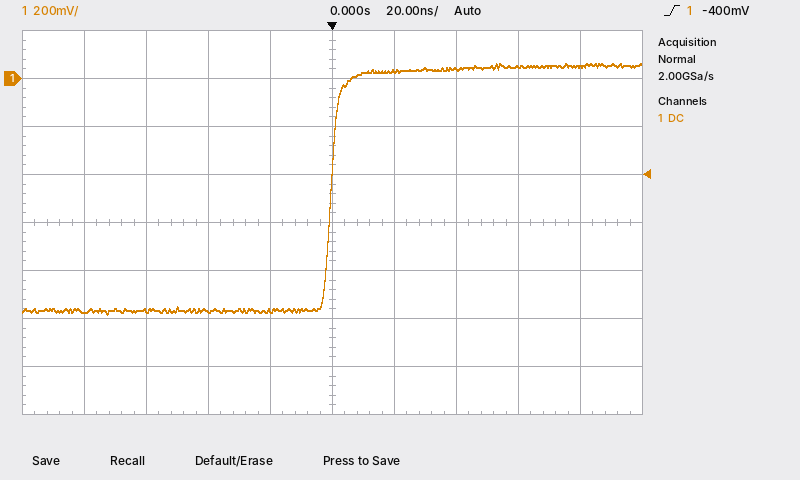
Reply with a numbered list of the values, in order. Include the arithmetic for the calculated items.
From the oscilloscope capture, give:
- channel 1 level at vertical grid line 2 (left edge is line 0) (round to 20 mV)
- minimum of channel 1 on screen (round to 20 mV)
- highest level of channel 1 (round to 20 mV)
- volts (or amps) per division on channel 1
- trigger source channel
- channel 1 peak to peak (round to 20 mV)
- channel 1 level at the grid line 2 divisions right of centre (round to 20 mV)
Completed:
1. -960 mV
2. -980 mV
3. 60 mV
4. 200 mV
5. channel 1
6. 60 mV − (-980 mV) = 1.04 V
7. 40 mV
